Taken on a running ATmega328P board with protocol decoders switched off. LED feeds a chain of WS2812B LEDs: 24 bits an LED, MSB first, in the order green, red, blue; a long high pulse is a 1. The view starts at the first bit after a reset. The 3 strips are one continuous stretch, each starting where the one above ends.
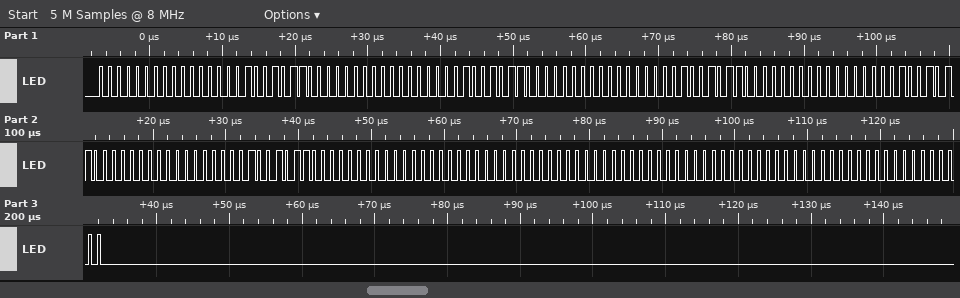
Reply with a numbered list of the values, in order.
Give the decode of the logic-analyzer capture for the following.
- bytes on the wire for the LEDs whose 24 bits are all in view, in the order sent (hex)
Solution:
1. 00 00 96 00 00 96 00 00 96 00 00 96 00 00 96 00 00 00 00 00 00 00 00 00
